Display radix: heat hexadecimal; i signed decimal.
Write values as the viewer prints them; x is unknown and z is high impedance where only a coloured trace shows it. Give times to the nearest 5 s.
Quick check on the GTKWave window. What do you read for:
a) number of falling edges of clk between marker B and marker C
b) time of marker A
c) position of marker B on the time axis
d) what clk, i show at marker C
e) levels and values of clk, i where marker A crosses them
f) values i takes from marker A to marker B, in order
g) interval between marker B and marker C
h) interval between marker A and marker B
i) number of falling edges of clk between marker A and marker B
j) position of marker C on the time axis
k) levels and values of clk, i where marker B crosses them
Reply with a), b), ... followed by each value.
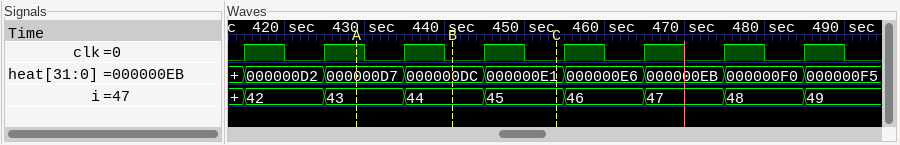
a) 1
b) 430 s
c) 440 s
d) clk=0, i=45
e) clk=1, i=43
f) 43, 44
g) 15 s
h) 10 s
i) 2
j) 455 s
k) clk=0, i=44
